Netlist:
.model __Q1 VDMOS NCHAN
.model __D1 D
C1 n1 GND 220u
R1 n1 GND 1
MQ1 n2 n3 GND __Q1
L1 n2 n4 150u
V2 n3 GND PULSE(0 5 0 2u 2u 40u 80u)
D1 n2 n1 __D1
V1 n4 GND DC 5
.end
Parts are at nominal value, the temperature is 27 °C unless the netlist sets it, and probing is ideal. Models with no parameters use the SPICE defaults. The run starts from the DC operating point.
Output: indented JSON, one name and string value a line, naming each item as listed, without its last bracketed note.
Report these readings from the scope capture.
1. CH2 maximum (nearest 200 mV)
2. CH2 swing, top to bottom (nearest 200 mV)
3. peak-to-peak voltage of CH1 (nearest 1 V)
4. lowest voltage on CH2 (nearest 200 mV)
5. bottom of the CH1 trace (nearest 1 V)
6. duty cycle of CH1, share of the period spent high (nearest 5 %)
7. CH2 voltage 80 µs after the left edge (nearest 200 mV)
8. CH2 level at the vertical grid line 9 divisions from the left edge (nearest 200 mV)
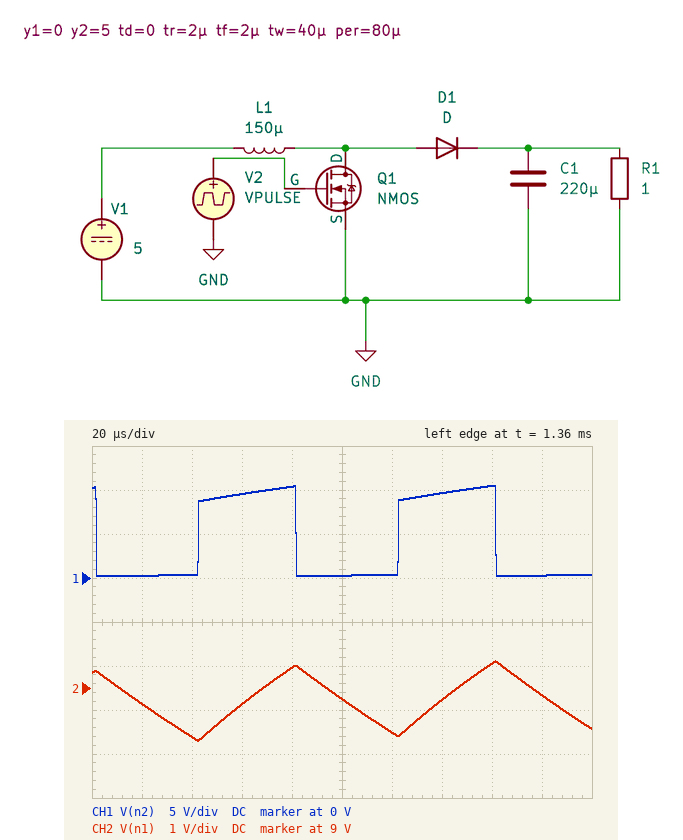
{
  "CH2 maximum": "9.6 V",
  "CH2 swing, top to bottom": "1.8 V",
  "peak-to-peak voltage of CH1": "10 V",
  "lowest voltage on CH2": "7.8 V",
  "bottom of the CH1 trace": "0 V",
  "duty cycle of CH1, share of the period spent high": "50 %",
  "CH2 voltage 80 µs after the left edge": "9.4 V",
  "CH2 level at the vertical grid line 9 divisions from the left edge": "8.8 V"
}
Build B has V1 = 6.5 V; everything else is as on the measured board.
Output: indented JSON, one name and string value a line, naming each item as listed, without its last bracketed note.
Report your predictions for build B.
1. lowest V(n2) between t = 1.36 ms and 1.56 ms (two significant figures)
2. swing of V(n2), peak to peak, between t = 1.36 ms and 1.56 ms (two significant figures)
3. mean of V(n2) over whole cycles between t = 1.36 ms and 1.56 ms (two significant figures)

{
  "lowest V(n2) between t = 1.36 ms and 1.56 ms": "370 mV",
  "swing of V(n2), peak to peak, between t = 1.36 ms and 1.56 ms": "13 V",
  "mean of V(n2) over whole cycles between t = 1.36 ms and 1.56 ms": "6.3 V"
}
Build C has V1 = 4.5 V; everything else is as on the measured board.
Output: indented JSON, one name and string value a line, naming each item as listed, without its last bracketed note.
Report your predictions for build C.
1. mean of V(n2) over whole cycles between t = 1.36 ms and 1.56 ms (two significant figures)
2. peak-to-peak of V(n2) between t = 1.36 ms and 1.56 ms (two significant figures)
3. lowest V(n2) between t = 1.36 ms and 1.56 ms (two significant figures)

{
  "mean of V(n2) over whole cycles between t = 1.36 ms and 1.56 ms": "4.4 V",
  "peak-to-peak of V(n2) between t = 1.36 ms and 1.56 ms": "9.2 V",
  "lowest V(n2) between t = 1.36 ms and 1.56 ms": "240 mV"
}
